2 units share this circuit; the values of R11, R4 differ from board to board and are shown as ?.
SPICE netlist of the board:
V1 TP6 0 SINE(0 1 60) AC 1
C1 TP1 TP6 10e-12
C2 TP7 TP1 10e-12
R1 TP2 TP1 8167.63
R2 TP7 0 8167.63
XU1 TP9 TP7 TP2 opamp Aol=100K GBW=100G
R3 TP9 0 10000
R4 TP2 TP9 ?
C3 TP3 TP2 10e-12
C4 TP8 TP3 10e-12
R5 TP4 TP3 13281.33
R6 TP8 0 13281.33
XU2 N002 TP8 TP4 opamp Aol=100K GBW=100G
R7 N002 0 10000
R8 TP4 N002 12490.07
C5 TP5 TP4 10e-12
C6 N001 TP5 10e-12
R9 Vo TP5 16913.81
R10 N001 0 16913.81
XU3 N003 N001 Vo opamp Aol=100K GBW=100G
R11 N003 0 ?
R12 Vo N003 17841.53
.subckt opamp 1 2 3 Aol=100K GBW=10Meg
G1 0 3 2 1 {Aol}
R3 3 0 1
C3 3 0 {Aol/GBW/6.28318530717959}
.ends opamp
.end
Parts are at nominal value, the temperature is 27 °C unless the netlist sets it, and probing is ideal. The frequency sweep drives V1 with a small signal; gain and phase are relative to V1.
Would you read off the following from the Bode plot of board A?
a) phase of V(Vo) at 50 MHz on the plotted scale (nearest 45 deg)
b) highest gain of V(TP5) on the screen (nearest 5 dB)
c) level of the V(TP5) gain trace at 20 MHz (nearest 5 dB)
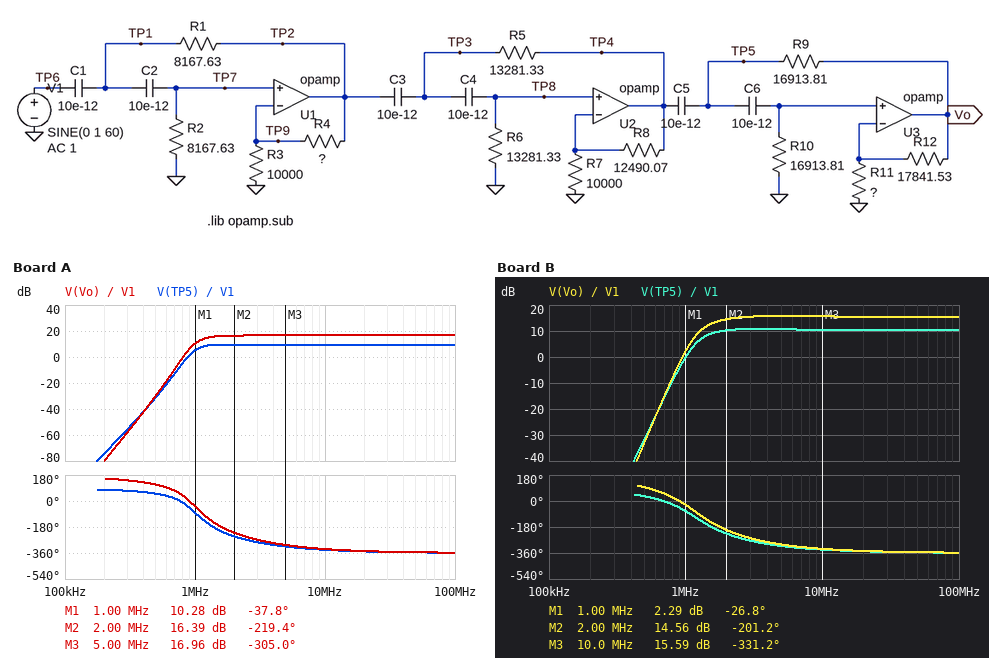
-360 deg
10 dB
10 dB
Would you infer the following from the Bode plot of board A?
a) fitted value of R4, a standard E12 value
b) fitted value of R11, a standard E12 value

2.7 kΩ
12 kΩ
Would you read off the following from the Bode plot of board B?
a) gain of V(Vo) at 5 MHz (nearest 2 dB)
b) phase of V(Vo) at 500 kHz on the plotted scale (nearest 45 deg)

16 dB
90 deg
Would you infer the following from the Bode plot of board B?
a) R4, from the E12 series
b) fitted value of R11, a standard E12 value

4.7 kΩ
22 kΩ
